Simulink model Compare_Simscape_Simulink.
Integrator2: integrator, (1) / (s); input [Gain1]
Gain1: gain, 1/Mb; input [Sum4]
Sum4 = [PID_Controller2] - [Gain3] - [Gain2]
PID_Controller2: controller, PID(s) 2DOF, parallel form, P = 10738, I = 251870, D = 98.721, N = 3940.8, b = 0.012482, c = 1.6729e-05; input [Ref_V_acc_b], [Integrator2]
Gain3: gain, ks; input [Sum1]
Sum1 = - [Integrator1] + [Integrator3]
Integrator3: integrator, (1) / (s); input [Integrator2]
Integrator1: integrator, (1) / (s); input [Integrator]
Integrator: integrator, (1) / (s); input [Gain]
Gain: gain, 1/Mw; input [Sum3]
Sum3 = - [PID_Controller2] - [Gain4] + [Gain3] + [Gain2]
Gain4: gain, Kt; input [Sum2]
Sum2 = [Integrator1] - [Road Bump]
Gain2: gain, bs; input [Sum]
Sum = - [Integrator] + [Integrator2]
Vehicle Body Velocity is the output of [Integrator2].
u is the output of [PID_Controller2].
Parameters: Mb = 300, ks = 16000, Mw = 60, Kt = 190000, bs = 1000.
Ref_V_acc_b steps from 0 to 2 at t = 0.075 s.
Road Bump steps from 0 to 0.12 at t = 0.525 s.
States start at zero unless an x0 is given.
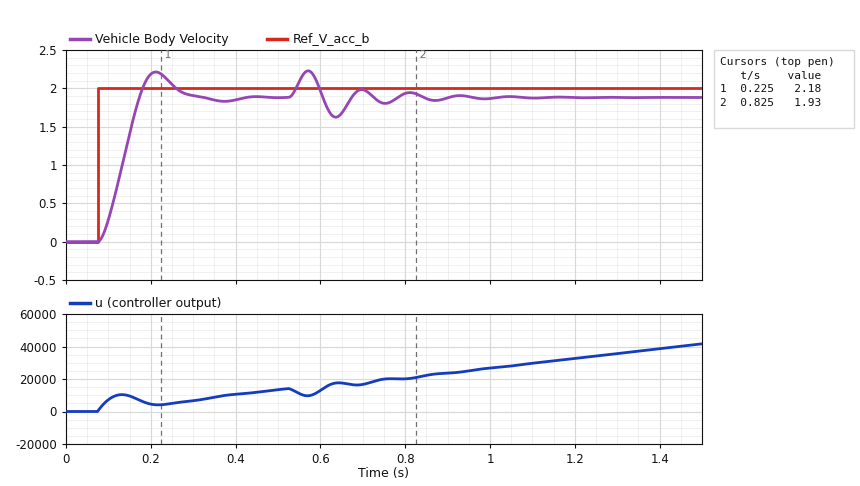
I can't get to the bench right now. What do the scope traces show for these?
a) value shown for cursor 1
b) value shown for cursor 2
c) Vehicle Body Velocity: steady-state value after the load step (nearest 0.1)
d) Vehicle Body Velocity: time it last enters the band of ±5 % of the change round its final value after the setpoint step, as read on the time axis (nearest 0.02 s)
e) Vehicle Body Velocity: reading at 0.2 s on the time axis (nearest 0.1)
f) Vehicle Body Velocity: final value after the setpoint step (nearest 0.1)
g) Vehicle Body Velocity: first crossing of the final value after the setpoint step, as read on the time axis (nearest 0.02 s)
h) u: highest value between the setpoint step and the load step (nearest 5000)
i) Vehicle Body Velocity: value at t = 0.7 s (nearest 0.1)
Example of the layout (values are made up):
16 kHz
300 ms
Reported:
2.18
1.93
1.9
0.26 s
2.2
1.9
0.18 s
15000
2.0
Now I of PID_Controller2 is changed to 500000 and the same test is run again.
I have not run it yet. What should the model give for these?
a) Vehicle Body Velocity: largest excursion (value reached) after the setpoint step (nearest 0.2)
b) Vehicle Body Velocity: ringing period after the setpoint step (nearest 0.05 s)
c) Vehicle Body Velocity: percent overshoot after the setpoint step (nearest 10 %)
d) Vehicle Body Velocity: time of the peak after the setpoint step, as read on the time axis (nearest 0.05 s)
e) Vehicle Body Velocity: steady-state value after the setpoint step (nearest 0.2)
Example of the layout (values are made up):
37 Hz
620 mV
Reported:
2.6
0.15 s
40 %
0.20 s
2.0
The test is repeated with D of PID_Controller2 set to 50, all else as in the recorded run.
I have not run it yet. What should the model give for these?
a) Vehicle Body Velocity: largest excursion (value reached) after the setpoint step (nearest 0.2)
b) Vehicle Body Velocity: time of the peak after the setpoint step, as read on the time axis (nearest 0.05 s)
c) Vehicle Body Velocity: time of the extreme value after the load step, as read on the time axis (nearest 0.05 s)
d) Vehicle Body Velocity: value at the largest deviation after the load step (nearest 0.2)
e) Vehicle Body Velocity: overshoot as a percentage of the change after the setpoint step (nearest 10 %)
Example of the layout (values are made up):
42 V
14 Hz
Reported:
2.2
0.20 s
0.55 s
2.2
20 %
